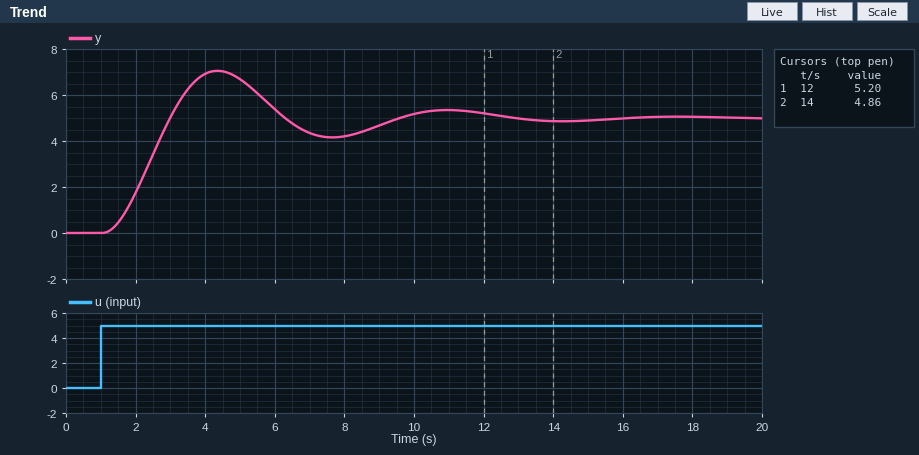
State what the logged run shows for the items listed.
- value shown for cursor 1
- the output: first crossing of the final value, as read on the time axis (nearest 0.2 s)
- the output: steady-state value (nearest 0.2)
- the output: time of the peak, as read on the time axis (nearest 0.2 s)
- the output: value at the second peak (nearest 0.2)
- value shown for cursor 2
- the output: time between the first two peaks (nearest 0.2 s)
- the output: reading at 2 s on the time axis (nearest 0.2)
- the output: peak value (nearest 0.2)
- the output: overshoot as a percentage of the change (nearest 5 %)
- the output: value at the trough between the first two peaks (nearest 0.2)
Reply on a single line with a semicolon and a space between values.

5.20; 3.0 s; 5.0; 4.4 s; 5.4; 4.86; 6.6 s; 1.8; 7.0; 40 %; 4.2
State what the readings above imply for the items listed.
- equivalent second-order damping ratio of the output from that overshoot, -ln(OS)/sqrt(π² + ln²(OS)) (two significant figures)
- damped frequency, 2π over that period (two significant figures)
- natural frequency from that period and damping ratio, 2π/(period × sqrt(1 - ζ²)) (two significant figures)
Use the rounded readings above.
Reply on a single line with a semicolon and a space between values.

0.28; 0.95 rad/s; 0.99 rad/s
